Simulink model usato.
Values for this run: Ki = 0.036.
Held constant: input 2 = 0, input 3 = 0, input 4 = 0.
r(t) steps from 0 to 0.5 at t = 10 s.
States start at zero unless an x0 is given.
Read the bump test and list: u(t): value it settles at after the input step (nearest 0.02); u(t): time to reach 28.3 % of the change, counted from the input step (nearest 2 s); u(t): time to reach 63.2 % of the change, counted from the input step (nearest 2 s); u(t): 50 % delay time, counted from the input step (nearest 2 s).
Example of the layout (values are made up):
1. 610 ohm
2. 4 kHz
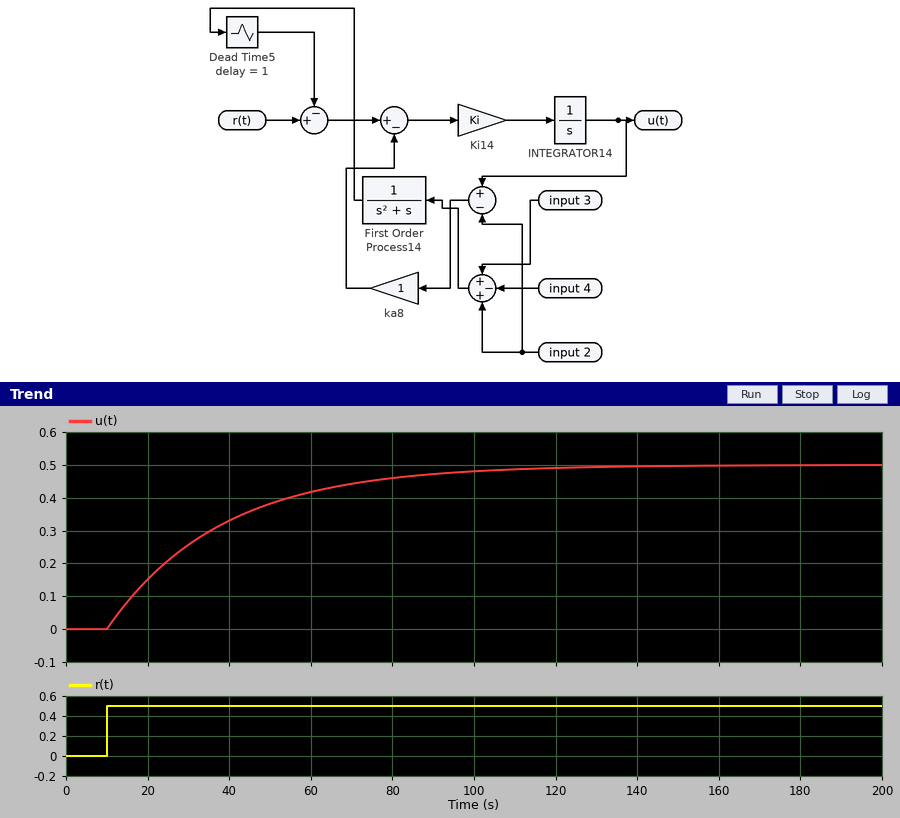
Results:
1. 0.50
2. 10 s
3. 28 s
4. 20 s
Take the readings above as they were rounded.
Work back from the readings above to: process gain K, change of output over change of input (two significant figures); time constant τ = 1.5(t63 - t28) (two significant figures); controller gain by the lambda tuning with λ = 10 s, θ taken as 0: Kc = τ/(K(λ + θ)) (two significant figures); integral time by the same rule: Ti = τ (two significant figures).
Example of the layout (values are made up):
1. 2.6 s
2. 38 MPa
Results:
1. 1.0
2. 27 s
3. 2.7
4. 27 s
